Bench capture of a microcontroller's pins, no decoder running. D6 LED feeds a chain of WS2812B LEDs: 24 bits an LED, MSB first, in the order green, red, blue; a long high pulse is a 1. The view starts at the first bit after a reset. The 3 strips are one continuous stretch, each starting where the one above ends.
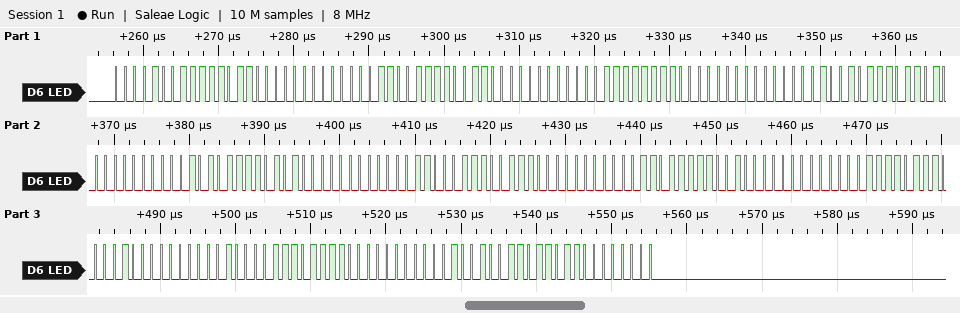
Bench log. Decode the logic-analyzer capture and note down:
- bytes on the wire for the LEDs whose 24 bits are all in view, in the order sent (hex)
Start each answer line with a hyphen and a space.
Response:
- 09 F6 00 0C F3 00 0F F0 00 12 ED 00 15 EA 00 18 E7 00 1B E4 00 1E E1 00 21 DE 00 24 DB 00
